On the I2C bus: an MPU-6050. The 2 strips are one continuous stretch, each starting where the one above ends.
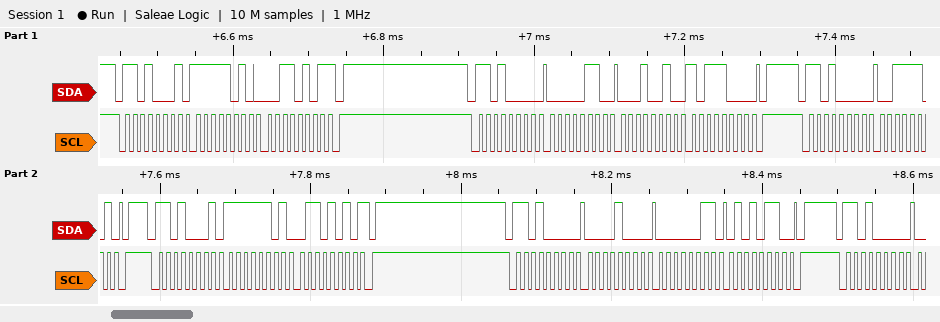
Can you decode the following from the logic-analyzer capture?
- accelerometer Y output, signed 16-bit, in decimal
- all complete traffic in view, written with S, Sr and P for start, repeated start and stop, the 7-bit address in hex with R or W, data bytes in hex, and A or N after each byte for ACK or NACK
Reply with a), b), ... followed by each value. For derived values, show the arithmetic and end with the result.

a) 0xFD6A = -662
b) S 68R A FA A 35 N P S 68W A 06 A 12 A B8 A P S 68W A 3D A P S 68R A FD A 6A N P S 68W A 08 A 03 A 56 A P S 68W A
